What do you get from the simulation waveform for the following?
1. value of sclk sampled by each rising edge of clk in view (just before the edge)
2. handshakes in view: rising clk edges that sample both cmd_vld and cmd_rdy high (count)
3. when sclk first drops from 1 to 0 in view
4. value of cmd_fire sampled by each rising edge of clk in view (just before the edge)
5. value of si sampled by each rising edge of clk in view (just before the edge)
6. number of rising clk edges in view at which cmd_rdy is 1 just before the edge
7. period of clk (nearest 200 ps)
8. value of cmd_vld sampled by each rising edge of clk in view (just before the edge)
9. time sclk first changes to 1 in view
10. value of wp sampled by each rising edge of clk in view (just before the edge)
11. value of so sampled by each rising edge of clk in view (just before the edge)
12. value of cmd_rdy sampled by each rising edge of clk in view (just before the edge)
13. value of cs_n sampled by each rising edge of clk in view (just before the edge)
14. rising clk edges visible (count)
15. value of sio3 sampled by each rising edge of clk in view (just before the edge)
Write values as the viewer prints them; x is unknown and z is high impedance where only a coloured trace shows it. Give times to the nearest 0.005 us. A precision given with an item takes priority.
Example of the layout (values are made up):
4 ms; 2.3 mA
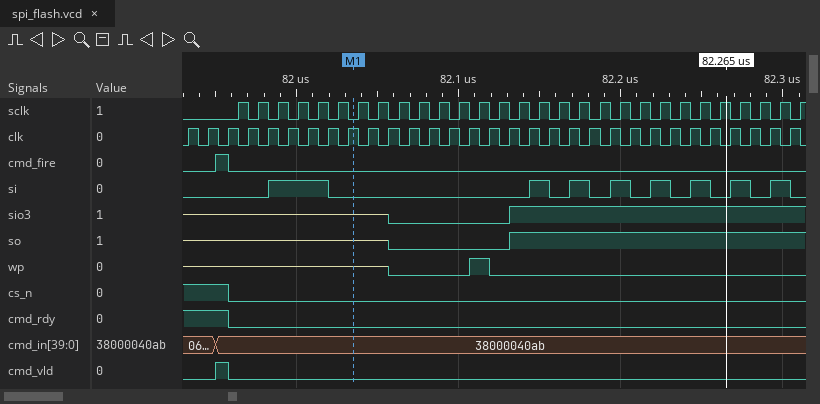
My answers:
0 0 0 1 1 1 1 1 1 1 1 1 1 1 1 1 1 1 1 1 1 1 1 1 1 1 1 1 1 1 1; 1; 81.97 us; 0 0 1 0 0 0 0 0 0 0 0 0 0 0 0 0 0 0 0 0 0 0 0 0 0 0 0 0 0 0 0; 0 0 0 0 0 1 1 1 0 0 0 0 0 0 0 0 0 0 1 0 1 0 1 0 1 0 1 0 1 0 1; 3; 12400 ps; 0 0 1 0 0 0 0 0 0 0 0 0 0 0 0 0 0 0 0 0 0 0 0 0 0 0 0 0 0 0 0; 81.965 us; z z z z z z z z z z z 0 0 0 0 1 0 0 0 0 0 0 0 0 0 0 0 0 0 0 0; z z z z z z z z z z z 0 0 0 0 0 0 1 1 1 1 1 1 1 1 1 1 1 1 1 1; 1 1 1 0 0 0 0 0 0 0 0 0 0 0 0 0 0 0 0 0 0 0 0 0 0 0 0 0 0 0 0; 1 1 1 0 0 0 0 0 0 0 0 0 0 0 0 0 0 0 0 0 0 0 0 0 0 0 0 0 0 0 0; 31; z z z z z z z z z z z 0 0 0 0 0 0 1 1 1 1 1 1 1 1 1 1 1 1 1 1
